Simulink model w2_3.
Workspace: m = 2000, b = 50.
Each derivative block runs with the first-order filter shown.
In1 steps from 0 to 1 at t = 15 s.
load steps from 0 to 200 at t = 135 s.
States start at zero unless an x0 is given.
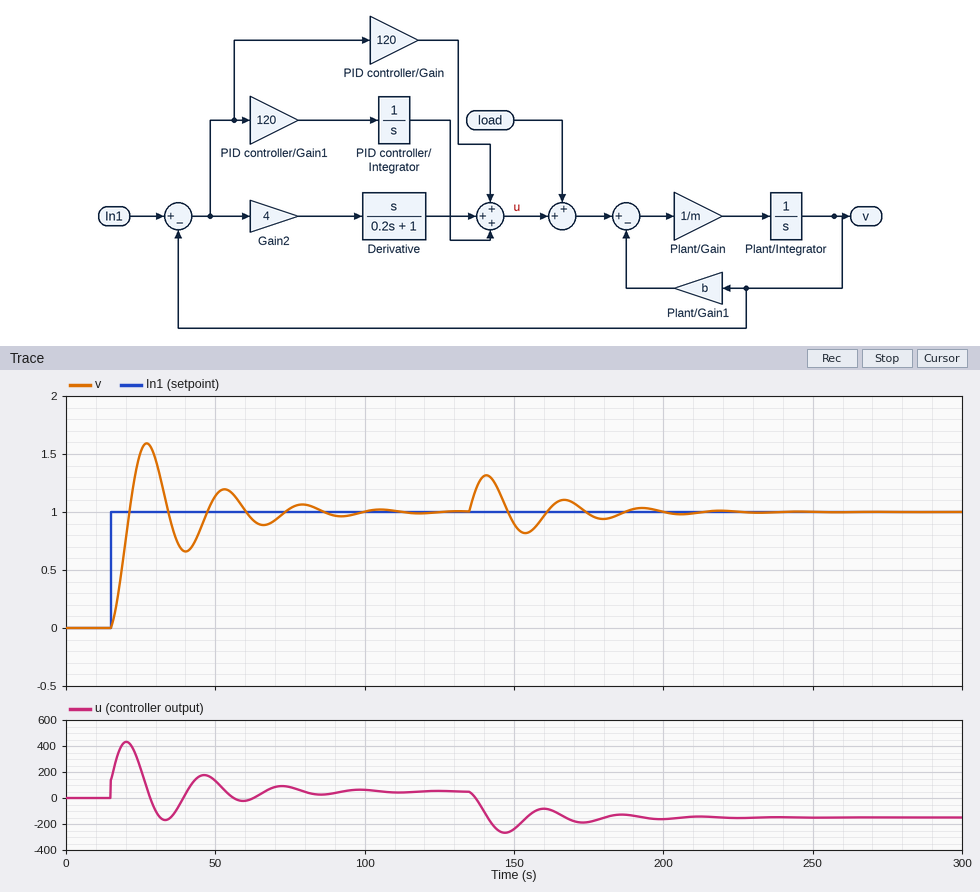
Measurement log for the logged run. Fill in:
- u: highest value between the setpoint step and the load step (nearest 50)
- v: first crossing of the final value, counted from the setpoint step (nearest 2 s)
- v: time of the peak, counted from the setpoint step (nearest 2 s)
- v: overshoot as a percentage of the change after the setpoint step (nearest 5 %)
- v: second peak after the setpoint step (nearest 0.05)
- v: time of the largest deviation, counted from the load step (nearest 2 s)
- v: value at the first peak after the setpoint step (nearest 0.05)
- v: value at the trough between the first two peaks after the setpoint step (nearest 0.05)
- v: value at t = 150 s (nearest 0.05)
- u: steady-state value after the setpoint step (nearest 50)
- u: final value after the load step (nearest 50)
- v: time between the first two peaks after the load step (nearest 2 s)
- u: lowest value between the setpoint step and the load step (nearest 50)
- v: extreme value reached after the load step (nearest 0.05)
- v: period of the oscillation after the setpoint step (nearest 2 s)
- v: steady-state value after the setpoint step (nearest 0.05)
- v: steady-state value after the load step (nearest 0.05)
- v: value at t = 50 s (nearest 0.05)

450
6 s
12 s
60 %
1.20
6 s
1.60
0.65
0.90
50
-150
26 s
-150
1.30
26 s
1.00
1.00
1.15
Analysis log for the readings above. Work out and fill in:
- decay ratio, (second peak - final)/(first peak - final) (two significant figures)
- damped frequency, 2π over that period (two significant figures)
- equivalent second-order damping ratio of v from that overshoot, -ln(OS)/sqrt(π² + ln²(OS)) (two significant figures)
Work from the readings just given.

0.33
0.24 rad/s
0.16
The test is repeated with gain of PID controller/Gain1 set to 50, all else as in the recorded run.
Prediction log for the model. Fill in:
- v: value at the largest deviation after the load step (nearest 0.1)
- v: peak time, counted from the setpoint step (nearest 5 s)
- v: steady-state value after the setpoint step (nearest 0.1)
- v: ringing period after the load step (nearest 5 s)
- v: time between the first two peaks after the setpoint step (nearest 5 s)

1.4
20 s
1.0
40 s
40 s
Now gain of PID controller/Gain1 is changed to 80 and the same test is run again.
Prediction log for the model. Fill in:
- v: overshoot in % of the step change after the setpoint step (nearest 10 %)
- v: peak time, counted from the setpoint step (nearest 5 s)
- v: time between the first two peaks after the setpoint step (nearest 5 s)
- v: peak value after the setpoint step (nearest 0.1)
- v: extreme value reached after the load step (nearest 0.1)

50 %
15 s
30 s
1.5
1.4
